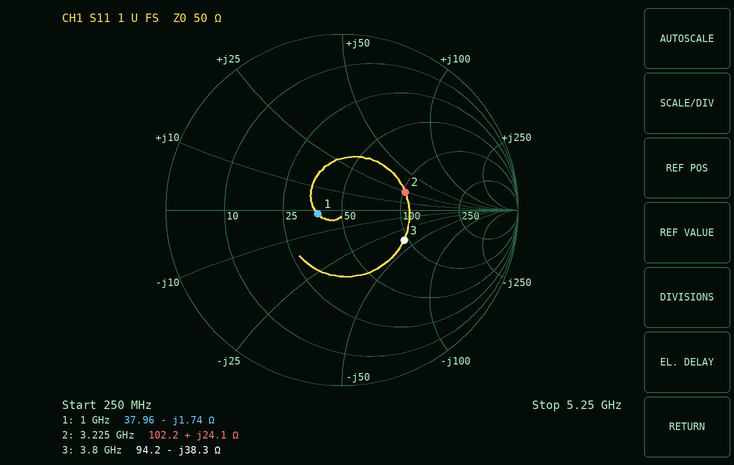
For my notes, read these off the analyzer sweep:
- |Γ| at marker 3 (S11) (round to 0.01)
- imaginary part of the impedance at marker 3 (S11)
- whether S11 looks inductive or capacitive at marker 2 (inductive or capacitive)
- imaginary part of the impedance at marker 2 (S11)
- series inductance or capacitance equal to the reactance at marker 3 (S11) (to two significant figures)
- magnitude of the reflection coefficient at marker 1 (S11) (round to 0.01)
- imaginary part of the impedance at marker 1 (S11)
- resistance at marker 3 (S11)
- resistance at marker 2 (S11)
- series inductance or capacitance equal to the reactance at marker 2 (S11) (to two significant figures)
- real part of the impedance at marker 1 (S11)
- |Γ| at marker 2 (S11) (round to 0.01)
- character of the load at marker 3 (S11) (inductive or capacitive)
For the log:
0.39
-38.3 Ω
inductive
+24.1 Ω
1.1 pF
0.14
-1.74 Ω
94.2 Ω
102.2 Ω
1.2 nH
37.96 Ω
0.37
capacitive
